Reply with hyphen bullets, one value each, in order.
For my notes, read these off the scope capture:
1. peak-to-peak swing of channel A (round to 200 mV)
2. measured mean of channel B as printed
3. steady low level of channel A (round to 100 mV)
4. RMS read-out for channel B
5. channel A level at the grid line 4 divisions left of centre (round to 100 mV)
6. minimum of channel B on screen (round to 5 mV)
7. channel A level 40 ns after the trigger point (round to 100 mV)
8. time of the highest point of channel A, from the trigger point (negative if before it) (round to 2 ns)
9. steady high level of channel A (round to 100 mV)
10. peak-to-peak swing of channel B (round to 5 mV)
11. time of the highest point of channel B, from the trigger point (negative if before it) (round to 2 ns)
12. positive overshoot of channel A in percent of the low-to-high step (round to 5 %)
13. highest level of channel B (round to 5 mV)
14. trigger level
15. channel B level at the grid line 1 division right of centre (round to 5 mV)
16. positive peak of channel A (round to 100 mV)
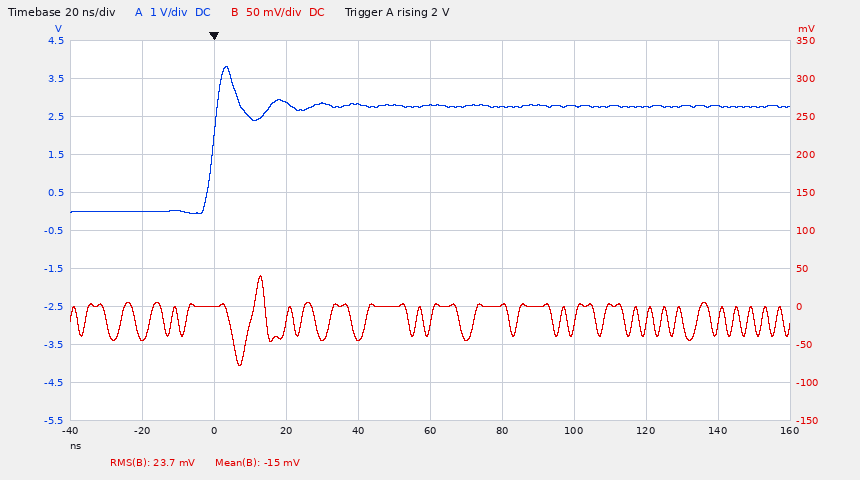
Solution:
- 3.8 V
- -15 mV
- 0.0 V
- 23.7 mV
- 0.0 V
- -80 mV
- 2.8 V
- +4 ns
- 2.8 V
- 120 mV
- +12 ns
- 40 %
- 40 mV
- 2 V
- 0 mV
- 3.8 V
